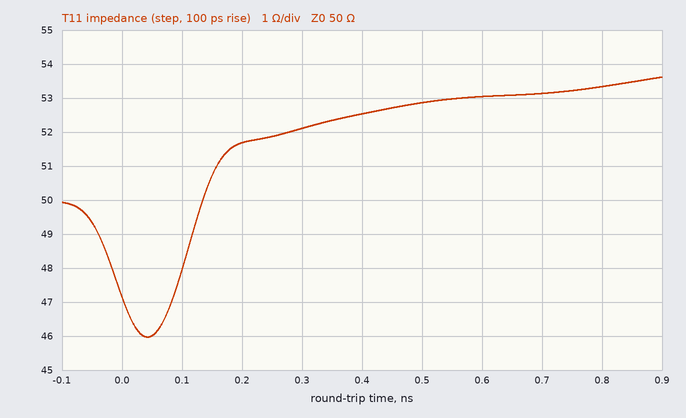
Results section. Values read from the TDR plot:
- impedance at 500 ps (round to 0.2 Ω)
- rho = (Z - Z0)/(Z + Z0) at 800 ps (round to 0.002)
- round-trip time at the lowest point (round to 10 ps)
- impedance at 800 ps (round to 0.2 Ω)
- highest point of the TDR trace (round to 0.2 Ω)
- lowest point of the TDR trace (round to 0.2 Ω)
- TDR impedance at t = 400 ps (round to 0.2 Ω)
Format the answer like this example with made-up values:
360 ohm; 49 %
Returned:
52.8 Ω; +0.032; 40 ps; 53.4 Ω; 53.6 Ω; 46.0 Ω; 52.6 Ω
